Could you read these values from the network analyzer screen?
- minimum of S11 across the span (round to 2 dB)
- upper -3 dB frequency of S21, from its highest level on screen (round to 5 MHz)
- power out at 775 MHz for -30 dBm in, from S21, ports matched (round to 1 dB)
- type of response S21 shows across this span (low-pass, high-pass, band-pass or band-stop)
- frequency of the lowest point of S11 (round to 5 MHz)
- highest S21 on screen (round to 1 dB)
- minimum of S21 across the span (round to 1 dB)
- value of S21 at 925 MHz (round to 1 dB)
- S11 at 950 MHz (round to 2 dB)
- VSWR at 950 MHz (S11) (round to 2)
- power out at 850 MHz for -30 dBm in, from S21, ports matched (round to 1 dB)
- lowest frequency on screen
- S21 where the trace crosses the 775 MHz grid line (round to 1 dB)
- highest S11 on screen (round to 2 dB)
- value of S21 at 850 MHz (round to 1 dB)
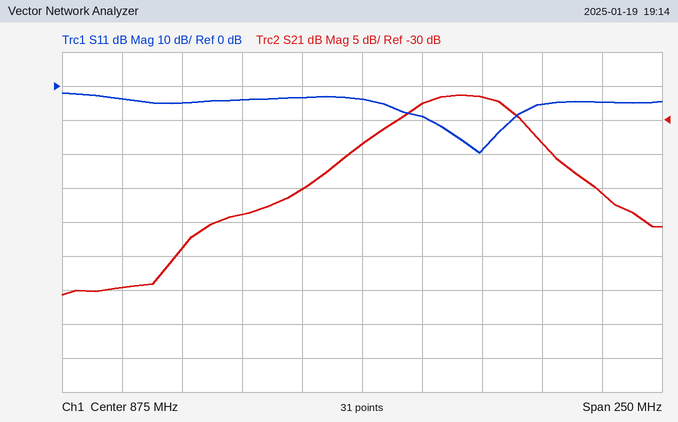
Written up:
-20 dB
940 MHz
-85 dBm
band-pass
925 MHz
-26 dB
-56 dB
-27 dB
-6 dB
4
-70 dBm
750 MHz
-55 dB
-2 dB
-40 dB
